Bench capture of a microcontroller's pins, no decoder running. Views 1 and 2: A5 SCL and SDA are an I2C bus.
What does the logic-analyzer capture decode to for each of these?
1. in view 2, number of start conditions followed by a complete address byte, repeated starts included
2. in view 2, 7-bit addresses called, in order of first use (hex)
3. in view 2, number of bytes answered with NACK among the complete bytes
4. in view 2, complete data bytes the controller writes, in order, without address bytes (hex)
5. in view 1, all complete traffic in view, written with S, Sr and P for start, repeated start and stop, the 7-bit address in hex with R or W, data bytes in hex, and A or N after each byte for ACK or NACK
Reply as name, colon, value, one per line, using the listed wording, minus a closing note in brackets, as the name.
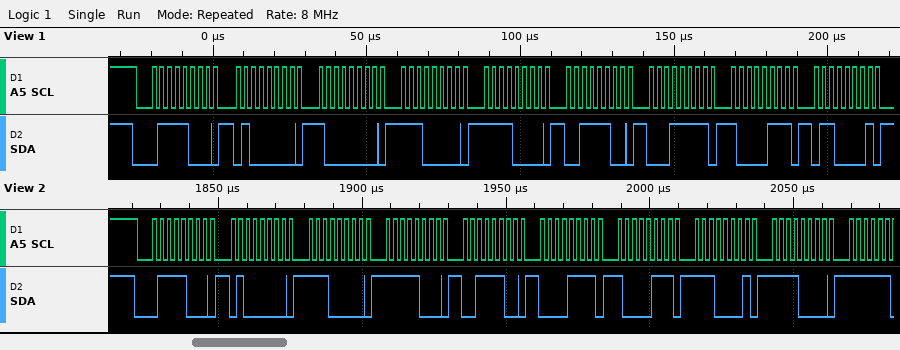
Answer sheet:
in view 2, number of start conditions followed by a complete address byte, repeated starts included: 1
in view 2, 7-bit addresses called, in order of first use: 0x3C
in view 2, number of bytes answered with NACK among the complete bytes: 0
in view 2, complete data bytes the controller writes, in order, without address bytes: 40 E0 F8 3C 0F 87 E1 F0
in view 1, all complete traffic in view, written with S, Sr and P for start, repeated start and stop, the 7-bit address in hex with R or W, data bytes in hex, and A or N after each byte for ACK or NACK: S 3CW A 40 A 80 A E0 A F0 A 3C A 1F A 87 A 61 A
